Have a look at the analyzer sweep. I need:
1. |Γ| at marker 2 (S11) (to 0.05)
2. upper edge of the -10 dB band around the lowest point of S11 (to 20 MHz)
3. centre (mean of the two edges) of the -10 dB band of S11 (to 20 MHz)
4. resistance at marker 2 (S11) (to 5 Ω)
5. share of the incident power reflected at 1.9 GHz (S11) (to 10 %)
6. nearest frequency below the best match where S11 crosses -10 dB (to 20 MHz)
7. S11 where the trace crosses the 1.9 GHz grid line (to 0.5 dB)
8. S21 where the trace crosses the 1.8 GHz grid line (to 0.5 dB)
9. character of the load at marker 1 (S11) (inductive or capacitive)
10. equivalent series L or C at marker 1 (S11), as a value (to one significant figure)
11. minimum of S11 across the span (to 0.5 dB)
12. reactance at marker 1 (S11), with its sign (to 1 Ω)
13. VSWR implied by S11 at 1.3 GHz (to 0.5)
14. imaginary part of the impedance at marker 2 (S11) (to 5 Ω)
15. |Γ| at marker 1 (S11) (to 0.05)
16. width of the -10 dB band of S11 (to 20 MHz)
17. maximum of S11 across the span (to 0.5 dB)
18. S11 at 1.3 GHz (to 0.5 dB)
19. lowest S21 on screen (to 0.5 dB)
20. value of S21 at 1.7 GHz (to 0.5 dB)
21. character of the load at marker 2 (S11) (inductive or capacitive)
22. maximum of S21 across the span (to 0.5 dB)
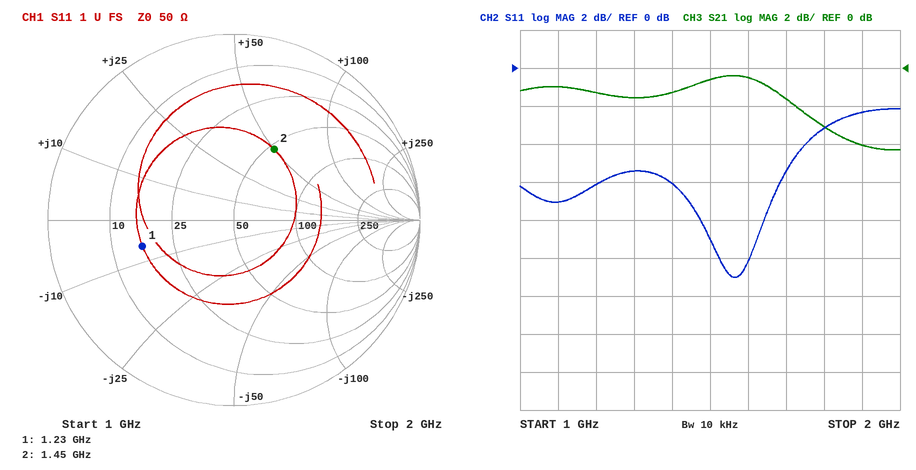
0.45
1.60 GHz
1.56 GHz
55 Ω
60 %
1.52 GHz
-2.5 dB
-3.0 dB
capacitive
20 pF
-11.0 dB
-6 Ω
3.5
+50 Ω
0.50
80 MHz
-2.0 dB
-5.5 dB
-4.5 dB
-1.5 dB
inductive
-0.5 dB
